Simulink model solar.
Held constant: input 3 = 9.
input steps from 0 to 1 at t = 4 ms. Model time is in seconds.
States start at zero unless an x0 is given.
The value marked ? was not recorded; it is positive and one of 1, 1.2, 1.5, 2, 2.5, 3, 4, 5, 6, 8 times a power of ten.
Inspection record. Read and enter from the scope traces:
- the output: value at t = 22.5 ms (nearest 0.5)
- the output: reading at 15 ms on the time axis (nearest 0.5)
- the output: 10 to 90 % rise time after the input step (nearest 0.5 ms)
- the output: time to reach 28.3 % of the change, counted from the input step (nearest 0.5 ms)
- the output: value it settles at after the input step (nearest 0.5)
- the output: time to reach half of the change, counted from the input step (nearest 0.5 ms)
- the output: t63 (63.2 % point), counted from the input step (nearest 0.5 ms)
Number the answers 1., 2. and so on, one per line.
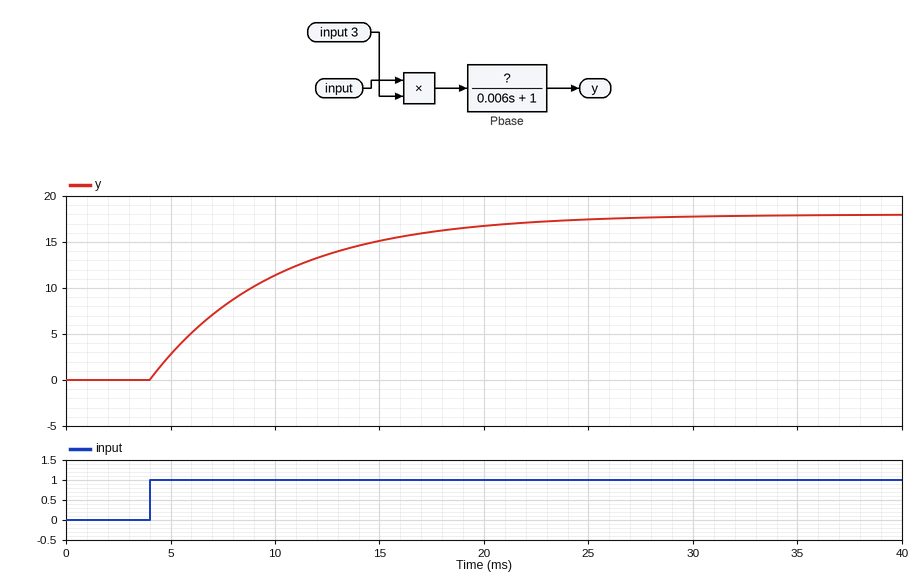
1. 17.0
2. 15.0
3. 13.0 ms
4. 2.0 ms
5. 18.0
6. 4.0 ms
7. 6.0 ms
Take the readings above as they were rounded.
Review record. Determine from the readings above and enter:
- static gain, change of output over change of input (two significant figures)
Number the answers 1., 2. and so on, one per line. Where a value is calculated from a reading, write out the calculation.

1. (18 - 0) / (1 - 0) = 18
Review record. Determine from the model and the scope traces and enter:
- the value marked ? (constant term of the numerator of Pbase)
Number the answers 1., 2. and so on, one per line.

1. 2
